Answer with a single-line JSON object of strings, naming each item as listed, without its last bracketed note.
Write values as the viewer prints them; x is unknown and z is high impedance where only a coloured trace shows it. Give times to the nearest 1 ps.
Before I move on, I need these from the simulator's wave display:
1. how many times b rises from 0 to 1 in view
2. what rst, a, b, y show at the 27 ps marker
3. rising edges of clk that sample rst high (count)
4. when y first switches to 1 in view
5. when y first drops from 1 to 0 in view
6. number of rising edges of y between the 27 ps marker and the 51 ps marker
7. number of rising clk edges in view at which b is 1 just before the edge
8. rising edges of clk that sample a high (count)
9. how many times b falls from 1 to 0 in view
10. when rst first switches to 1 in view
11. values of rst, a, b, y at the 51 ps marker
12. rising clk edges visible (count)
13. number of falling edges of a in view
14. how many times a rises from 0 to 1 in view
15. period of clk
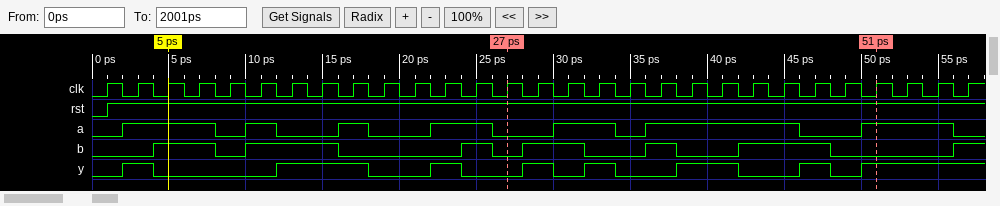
{"how many times b rises from 0 to 1 in view": "7", "what rst, a, b, y show at the 27 ps marker": "rst=1, a=0, b=0, y=0", "rising edges of clk that sample rst high": "28", "when y first switches to 1 in view": "2 ps", "when y first drops from 1 to 0 in view": "4 ps", "number of rising edges of y between the 27 ps marker and the 51 ps marker": "5", "number of rising clk edges in view at which b is 1 just before the edge": "13", "rising edges of clk that sample a high": "17", "how many times b falls from 1 to 0 in view": "6", "when rst first switches to 1 in view": "1 ps", "values of rst, a, b, y at the 51 ps marker": "rst=1, a=1, b=0, y=1", "rising clk edges visible": "29", "number of falling edges of a in view": "7", "how many times a rises from 0 to 1 in view": "7", "period of clk": "2 ps"}
